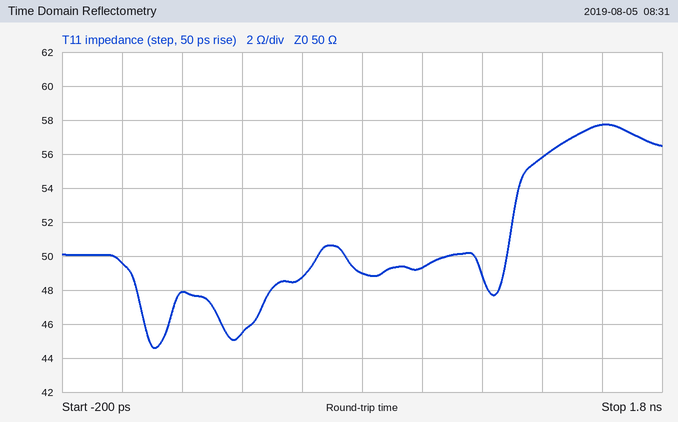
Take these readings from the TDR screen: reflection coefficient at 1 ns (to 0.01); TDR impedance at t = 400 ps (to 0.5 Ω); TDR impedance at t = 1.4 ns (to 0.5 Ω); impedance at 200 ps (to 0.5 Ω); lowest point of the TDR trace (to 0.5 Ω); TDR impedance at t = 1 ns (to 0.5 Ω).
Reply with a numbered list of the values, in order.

1. -0.01
2. 45.5 Ω
3. 56.0 Ω
4. 48.0 Ω
5. 44.5 Ω
6. 49.5 Ω
